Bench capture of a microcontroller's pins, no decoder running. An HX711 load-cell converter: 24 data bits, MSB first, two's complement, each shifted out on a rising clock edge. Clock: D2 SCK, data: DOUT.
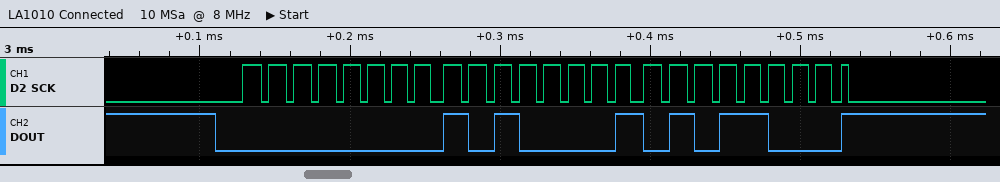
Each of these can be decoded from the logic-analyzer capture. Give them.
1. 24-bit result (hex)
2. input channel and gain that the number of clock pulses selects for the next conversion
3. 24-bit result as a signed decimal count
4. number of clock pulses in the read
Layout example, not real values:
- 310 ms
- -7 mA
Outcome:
- 0x00A158
- channel A, gain 128
- 41304
- 25
